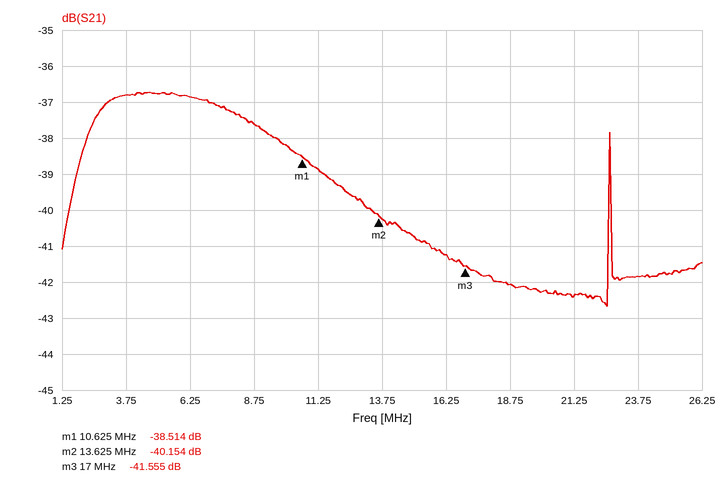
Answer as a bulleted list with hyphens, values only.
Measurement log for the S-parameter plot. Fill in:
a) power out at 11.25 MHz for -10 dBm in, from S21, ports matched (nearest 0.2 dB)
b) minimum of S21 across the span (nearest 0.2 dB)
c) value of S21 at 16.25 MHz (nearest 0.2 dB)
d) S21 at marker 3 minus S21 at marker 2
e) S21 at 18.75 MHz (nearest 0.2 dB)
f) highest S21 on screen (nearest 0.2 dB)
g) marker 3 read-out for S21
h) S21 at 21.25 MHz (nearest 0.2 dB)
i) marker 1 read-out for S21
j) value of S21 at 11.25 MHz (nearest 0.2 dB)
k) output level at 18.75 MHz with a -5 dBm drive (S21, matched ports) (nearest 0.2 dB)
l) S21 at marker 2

- -48.8 dBm
- -42.6 dB
- -41.2 dB
- -1.401 dB
- -42.0 dB
- -36.8 dB
- -41.555 dB
- -42.4 dB
- -38.514 dB
- -38.8 dB
- -47.0 dBm
- -40.154 dB
